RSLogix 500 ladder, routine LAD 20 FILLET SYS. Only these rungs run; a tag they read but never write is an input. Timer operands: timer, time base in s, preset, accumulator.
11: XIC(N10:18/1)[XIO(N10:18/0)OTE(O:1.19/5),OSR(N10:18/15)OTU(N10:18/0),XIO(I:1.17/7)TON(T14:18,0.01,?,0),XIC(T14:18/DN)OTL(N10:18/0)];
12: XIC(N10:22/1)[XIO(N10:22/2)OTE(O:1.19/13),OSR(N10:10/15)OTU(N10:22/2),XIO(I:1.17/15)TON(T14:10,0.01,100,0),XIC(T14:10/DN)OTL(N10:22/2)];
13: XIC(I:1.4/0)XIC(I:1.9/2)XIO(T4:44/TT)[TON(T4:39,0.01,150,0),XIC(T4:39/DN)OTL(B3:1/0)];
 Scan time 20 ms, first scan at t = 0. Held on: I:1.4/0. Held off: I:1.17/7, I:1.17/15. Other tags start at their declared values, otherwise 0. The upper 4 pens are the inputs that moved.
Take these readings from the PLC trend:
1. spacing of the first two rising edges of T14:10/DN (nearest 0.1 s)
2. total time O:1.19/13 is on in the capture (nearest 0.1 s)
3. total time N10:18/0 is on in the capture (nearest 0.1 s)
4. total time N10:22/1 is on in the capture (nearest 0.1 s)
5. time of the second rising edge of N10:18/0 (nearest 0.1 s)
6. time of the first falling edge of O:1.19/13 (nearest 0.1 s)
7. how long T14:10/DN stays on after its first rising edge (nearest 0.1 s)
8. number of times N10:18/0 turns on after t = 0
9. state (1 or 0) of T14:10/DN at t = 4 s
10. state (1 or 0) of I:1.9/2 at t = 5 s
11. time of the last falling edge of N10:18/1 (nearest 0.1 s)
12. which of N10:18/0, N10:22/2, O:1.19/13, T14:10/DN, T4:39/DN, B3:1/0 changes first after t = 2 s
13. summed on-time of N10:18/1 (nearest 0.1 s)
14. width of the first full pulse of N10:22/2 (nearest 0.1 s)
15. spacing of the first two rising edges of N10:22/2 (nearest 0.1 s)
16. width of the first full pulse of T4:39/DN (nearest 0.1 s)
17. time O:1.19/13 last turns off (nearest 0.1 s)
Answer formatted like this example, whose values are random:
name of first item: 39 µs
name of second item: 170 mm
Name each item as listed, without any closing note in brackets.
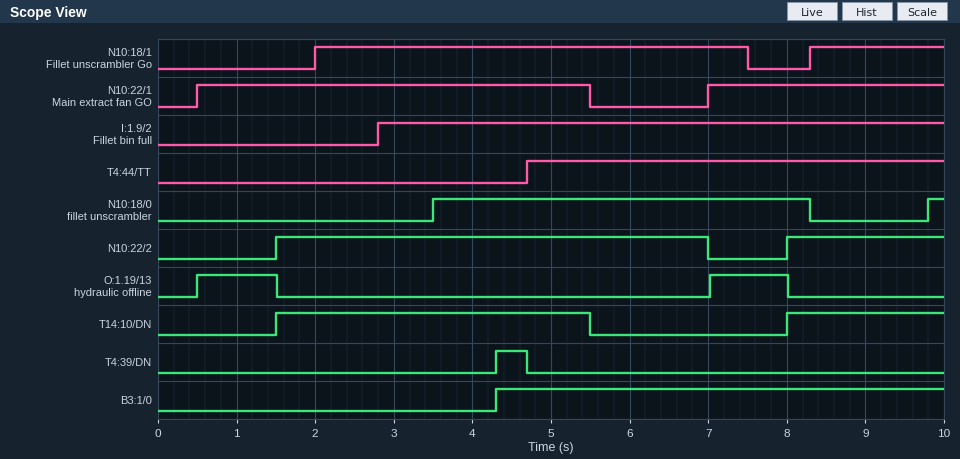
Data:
spacing of the first two rising edges of T14:10/DN: 6.5 s
total time O:1.19/13 is on in the capture: 2.0 s
total time N10:18/0 is on in the capture: 5.0 s
total time N10:22/1 is on in the capture: 8.0 s
time of the second rising edge of N10:18/0: 9.8 s
time of the first falling edge of O:1.19/13: 1.5 s
how long T14:10/DN stays on after its first rising edge: 4.0 s
number of times N10:18/0 turns on after t = 0: 2
state (1 or 0) of T14:10/DN at t = 4 s: 1
state (1 or 0) of I:1.9/2 at t = 5 s: 1
time of the last falling edge of N10:18/1: 7.5 s
which of N10:18/0, N10:22/2, O:1.19/13, T14:10/DN, T4:39/DN, B3:1/0 changes first after t = 2 s: N10:18/0
summed on-time of N10:18/1: 7.2 s
width of the first full pulse of N10:22/2: 5.5 s
spacing of the first two rising edges of N10:22/2: 6.5 s
width of the first full pulse of T4:39/DN: 0.4 s
time O:1.19/13 last turns off: 8.0 s
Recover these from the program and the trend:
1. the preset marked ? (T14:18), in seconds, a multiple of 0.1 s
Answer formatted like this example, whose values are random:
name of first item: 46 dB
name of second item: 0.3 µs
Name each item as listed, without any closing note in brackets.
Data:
the preset marked ? (T14:18), in seconds, a multiple of 0.1 s: 1.5 s
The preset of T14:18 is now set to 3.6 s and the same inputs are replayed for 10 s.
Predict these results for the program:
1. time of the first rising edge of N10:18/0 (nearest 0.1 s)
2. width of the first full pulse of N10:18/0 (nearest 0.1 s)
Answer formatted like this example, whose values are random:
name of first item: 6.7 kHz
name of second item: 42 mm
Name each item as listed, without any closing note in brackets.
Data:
time of the first rising edge of N10:18/0: 5.6 s
width of the first full pulse of N10:18/0: 2.7 s
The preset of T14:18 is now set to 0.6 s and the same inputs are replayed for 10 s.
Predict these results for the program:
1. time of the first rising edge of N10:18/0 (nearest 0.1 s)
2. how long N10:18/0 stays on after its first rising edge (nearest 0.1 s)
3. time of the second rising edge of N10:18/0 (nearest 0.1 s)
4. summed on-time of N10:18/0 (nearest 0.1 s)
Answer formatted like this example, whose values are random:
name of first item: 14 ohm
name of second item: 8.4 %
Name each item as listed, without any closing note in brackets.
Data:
time of the first rising edge of N10:18/0: 2.6 s
how long N10:18/0 stays on after its first rising edge: 5.7 s
time of the second rising edge of N10:18/0: 8.9 s
summed on-time of N10:18/0: 6.8 s
